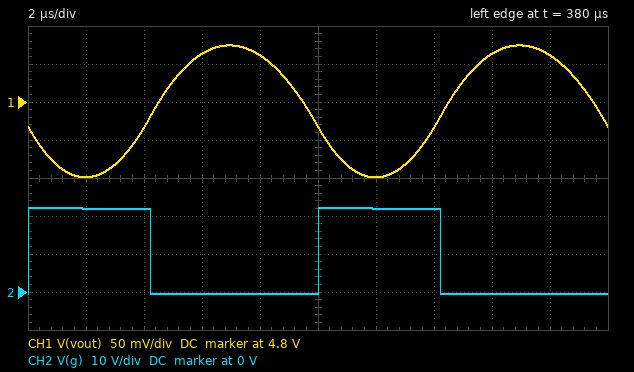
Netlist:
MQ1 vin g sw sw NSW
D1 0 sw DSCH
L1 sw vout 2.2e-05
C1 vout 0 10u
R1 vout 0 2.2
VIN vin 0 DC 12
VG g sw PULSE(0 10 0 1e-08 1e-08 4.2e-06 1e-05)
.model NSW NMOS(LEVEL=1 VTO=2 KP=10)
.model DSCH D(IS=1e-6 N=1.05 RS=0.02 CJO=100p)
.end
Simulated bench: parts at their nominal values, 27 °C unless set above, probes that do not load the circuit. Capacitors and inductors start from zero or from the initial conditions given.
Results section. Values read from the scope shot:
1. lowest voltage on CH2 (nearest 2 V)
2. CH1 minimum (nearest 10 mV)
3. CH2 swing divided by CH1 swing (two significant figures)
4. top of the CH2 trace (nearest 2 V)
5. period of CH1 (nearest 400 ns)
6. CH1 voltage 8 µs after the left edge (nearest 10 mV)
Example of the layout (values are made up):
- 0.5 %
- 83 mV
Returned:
- 0 V
- 4.70 V
- 130
- 22 V
- 10.0 µs
- 4.86 V
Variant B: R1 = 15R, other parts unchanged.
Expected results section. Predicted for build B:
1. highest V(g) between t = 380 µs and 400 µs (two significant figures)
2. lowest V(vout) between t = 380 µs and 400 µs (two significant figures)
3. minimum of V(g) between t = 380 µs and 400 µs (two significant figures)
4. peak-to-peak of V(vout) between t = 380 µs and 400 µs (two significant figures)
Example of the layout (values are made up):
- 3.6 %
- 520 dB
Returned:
- 22 V
- 6.3 V
- -400 mV
- 160 mV
